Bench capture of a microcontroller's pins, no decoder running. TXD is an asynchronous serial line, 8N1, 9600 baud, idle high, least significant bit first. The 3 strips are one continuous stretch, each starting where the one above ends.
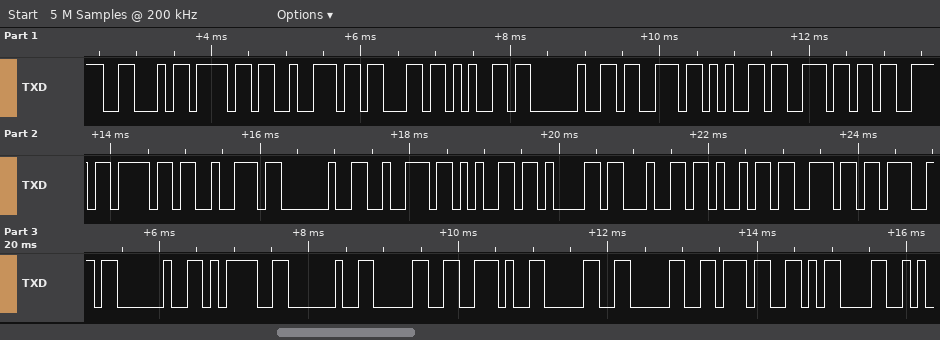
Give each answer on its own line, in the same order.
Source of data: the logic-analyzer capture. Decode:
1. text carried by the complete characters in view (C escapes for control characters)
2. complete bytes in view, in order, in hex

"Force sensor reading = 0.007\r"
0x46 0x6F 0x72 0x63 0x65 0x20 0x73 0x65 0x6E 0x73 0x6F 0x72 0x20 0x72 0x65 0x61 0x64 0x69 0x6E 0x67 0x20 0x3D 0x20 0x30 0x2E 0x30 0x30 0x37 0x0D
